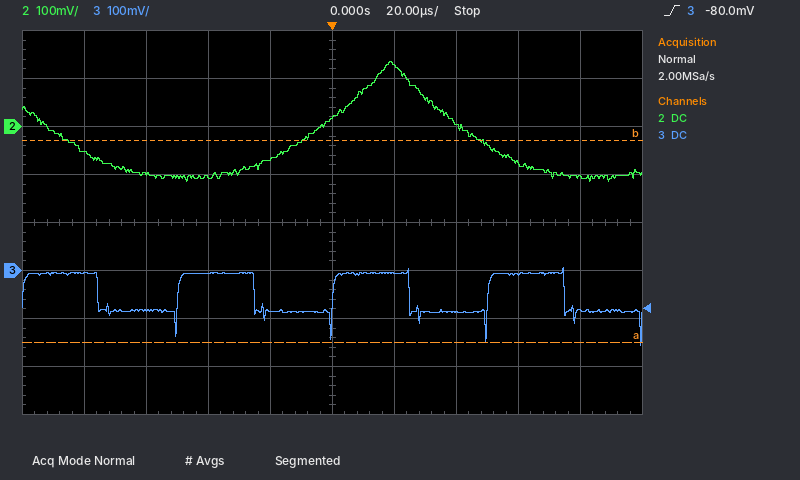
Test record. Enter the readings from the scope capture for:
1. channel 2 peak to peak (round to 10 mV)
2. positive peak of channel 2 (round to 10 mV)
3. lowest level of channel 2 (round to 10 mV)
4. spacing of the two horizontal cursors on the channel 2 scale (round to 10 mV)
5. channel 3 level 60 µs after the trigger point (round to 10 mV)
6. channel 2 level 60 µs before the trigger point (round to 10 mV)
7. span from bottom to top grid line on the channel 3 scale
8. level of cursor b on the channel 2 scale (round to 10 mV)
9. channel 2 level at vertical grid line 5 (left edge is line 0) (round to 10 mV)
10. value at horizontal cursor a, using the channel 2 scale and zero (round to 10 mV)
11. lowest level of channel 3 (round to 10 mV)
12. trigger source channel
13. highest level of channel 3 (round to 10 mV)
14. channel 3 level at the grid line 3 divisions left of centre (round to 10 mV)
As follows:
250 mV
140 mV
-110 mV
420 mV
-10 mV
-100 mV
800 mV
-30 mV
20 mV
-450 mV
-160 mV
channel 3
10 mV
-80 mV
